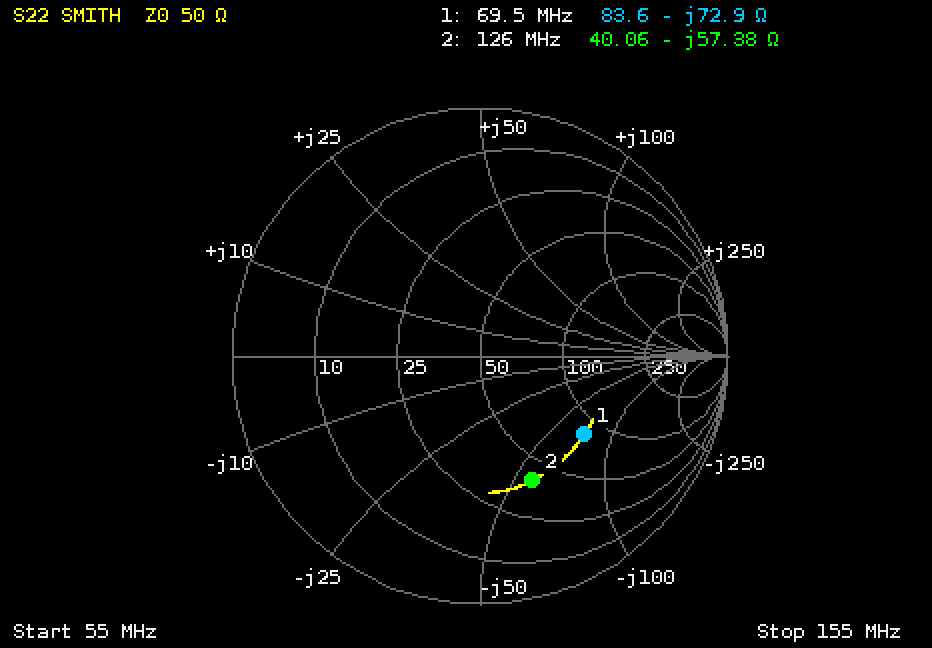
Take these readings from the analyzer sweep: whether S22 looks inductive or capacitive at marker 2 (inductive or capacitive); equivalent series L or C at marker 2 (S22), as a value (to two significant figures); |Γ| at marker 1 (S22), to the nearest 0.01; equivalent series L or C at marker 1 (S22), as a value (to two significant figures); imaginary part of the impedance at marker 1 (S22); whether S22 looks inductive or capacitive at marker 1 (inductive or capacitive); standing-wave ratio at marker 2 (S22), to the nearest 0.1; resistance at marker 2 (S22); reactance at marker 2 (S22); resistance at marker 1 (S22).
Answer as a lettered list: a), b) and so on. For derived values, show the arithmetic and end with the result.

a) capacitive
b) C = 1/(2π × 126 MHz × 57.38 Ω) ≈ 22 pF
c) 0.53
d) C = 1/(2π × 69.5 MHz × 72.9 Ω) ≈ 31 pF
e) -72.9 Ω
f) capacitive
g) 3.4
h) 40.06 Ω
i) -57.38 Ω
j) 83.6 Ω
